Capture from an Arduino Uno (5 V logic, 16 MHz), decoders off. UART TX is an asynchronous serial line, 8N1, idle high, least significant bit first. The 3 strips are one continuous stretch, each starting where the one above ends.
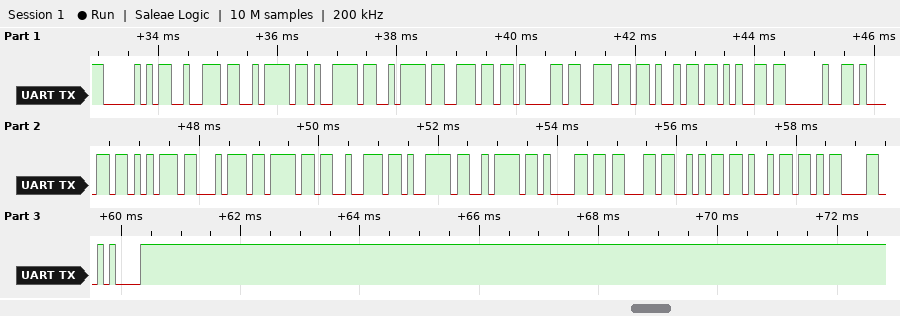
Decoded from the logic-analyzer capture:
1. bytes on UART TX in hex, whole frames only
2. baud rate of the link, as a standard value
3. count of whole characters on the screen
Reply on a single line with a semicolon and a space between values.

50 72 7A 79 7A 6E 61 6E 69 65 20 61 75 74 6F 72 79 7A 61 63 6A 69 0D 0A; 9600 baud; 24
